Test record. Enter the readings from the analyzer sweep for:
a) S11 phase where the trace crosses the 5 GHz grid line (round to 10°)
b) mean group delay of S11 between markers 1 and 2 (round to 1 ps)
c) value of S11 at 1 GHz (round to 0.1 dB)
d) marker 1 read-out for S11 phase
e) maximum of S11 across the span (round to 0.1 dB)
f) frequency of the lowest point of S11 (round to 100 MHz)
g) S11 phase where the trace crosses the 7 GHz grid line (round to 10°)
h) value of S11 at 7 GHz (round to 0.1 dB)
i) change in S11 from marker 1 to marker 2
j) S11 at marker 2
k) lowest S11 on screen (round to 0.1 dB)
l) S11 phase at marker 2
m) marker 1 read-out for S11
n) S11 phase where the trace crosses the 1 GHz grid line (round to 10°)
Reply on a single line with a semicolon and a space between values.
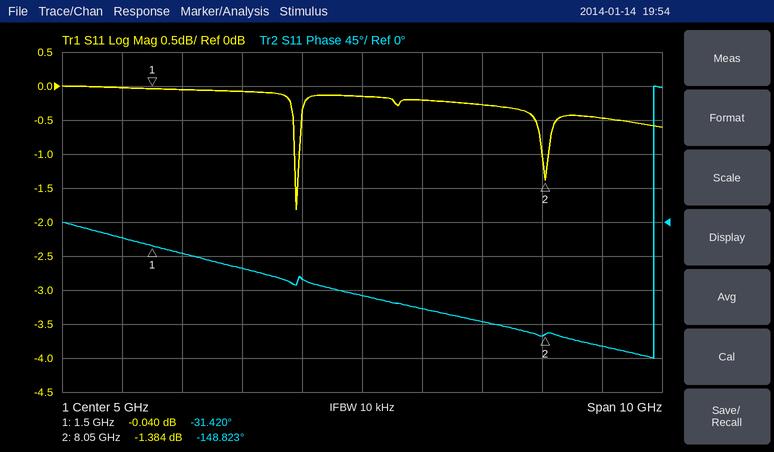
-100°; 50 ps; 0.0 dB; -31.420°; 0.0 dB; 3.9 GHz; -130°; -0.3 dB; -1.344 dB; -1.384 dB; -1.8 dB; -148.823°; -0.040 dB; -20°
